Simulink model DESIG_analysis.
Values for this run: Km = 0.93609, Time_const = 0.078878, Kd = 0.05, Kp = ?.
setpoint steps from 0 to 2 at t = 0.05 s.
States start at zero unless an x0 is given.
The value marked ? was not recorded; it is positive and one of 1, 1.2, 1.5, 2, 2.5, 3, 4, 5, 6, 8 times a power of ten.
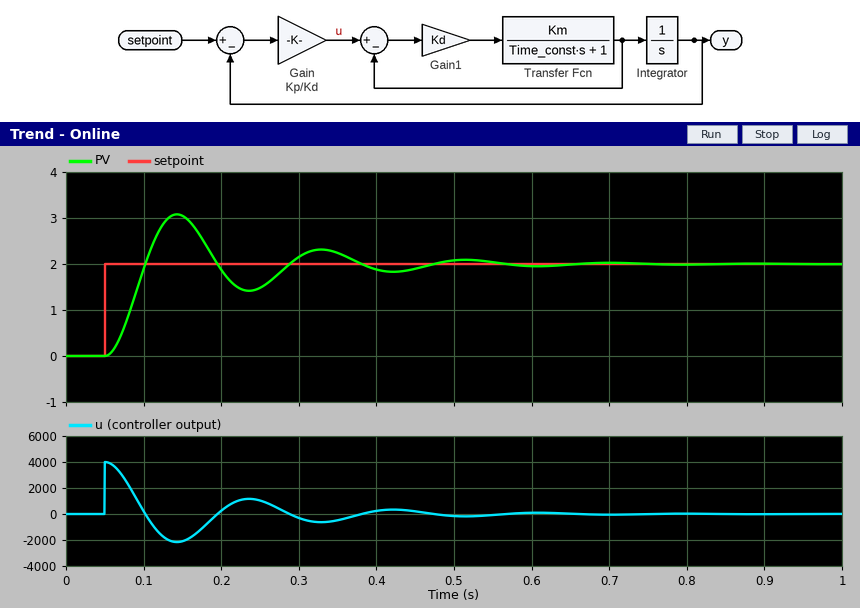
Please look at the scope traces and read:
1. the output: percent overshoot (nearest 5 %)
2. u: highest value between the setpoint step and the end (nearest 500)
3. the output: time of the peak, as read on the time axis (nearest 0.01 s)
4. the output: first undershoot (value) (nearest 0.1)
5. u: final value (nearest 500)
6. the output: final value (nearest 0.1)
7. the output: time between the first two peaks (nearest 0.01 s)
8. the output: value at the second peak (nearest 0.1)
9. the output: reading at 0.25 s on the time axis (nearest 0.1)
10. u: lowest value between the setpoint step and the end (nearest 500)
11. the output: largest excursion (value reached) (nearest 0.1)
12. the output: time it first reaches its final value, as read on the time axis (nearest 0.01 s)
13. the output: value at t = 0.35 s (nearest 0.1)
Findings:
55 %
4000
0.14 s
1.4
0
2.0
0.19 s
2.3
1.5
-2000
3.1
0.10 s
2.2
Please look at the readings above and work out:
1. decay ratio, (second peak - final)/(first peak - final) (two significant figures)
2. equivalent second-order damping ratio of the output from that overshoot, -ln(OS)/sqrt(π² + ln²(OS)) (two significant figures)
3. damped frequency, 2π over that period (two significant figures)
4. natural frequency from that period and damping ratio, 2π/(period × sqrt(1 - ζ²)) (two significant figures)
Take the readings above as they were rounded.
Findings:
0.27
0.19
33 rad/s
34 rad/s
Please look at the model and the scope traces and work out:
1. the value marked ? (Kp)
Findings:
100
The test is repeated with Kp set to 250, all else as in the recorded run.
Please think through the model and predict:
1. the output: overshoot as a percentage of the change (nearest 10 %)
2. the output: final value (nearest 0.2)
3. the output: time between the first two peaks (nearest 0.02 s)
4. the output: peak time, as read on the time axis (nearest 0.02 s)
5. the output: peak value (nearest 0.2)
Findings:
70 %
2.0
0.12 s
0.10 s
3.4
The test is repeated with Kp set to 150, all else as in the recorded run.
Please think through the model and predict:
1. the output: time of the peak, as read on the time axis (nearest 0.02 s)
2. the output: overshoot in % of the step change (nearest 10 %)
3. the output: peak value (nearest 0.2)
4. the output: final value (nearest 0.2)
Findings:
0.12 s
60 %
3.2
2.0
